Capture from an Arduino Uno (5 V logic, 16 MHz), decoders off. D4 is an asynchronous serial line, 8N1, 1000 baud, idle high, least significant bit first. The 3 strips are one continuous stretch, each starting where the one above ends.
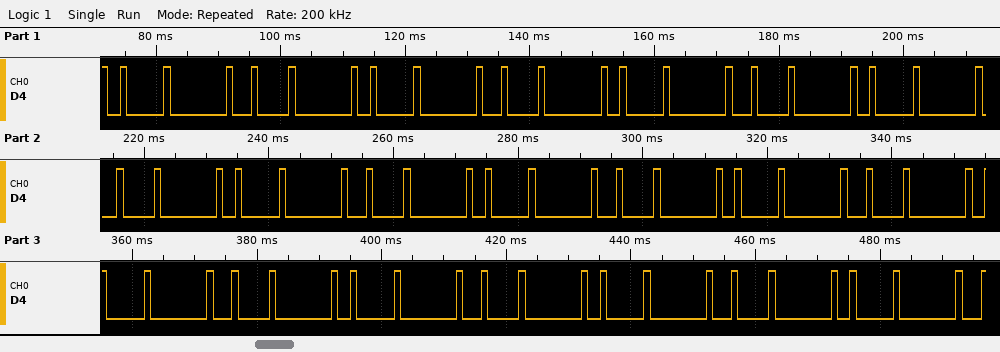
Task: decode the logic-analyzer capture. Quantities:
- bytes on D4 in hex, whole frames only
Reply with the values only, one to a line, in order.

0x02 0x00 0x04 0x00 0x02 0x00 0x04 0x00 0x02 0x00 0x04 0x00 0x02 0x00 0x04 0x00 0x02 0x00 0x04 0x00 0x02 0x00 0x04 0x00 0x02 0x00 0x04 0x00 0x02 0x00 0x04 0x00 0x02 0x00 0x04 0x00 0x02 0x00 0x04 0x00 0x02 0x00
